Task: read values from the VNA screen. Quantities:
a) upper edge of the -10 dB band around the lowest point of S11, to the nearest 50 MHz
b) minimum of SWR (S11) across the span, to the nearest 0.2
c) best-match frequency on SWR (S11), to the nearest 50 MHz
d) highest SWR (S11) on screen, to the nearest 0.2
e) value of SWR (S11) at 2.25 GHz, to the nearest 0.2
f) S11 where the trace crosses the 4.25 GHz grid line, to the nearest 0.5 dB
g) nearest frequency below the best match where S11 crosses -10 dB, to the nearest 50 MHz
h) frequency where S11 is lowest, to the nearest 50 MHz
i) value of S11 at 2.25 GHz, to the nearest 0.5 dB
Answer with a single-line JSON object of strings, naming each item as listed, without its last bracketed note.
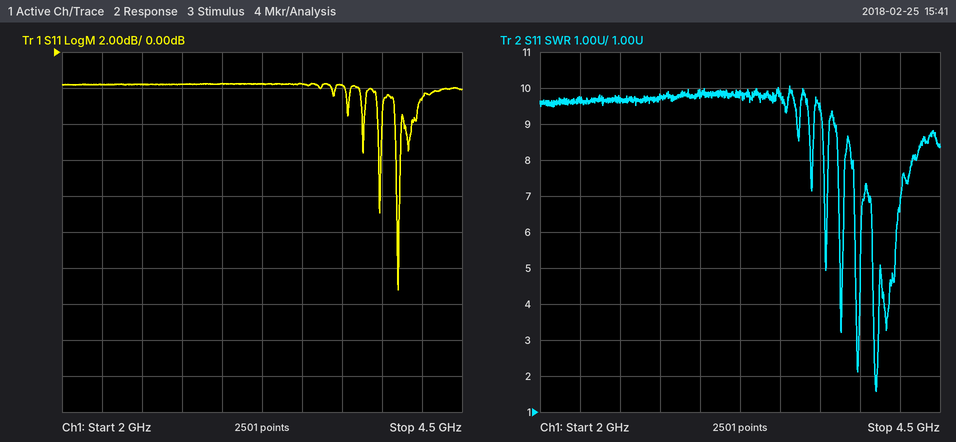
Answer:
{"upper edge of the -10 dB band around the lowest point of S11, to the nearest 50 MHz": "4.10 GHz", "minimum of SWR (S11) across the span, to the nearest 0.2": "1.6", "best-match frequency on SWR (S11), to the nearest 50 MHz": "4.10 GHz", "highest SWR (S11) on screen, to the nearest 0.2": "10.0", "value of SWR (S11) at 2.25 GHz, to the nearest 0.2": "9.6", "S11 where the trace crosses the 4.25 GHz grid line, to the nearest 0.5 dB": "-2.5 dB", "nearest frequency below the best match where S11 crosses -10 dB, to the nearest 50 MHz": "4.10 GHz", "frequency where S11 is lowest, to the nearest 50 MHz": "4.10 GHz", "value of S11 at 2.25 GHz, to the nearest 0.5 dB": "-2.0 dB"}
